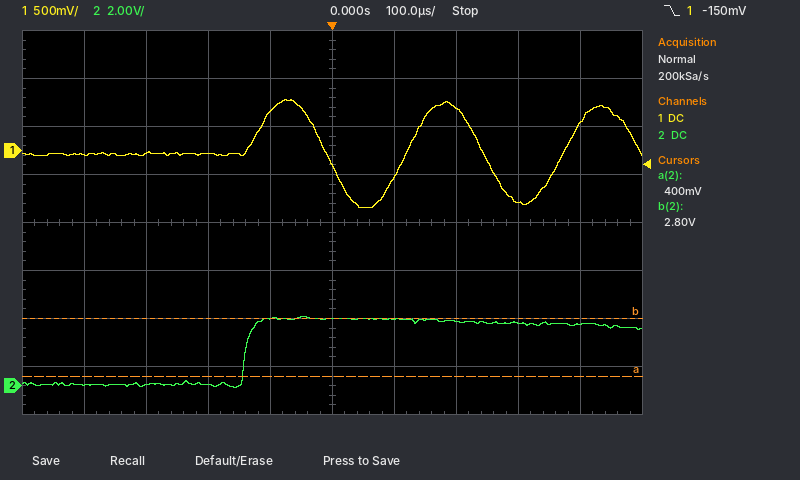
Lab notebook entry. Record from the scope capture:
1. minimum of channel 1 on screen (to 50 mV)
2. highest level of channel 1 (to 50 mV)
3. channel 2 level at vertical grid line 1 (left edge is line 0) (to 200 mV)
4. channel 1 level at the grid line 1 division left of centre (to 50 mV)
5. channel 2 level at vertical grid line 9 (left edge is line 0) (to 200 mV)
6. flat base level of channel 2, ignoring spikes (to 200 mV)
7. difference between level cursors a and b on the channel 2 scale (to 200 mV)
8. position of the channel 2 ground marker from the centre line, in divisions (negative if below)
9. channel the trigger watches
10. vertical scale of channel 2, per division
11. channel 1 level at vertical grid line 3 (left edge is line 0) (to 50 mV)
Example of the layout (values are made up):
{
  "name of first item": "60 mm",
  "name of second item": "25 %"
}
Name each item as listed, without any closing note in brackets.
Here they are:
{
  "minimum of channel 1 on screen": "-600 mV",
  "highest level of channel 1": "550 mV",
  "channel 2 level at vertical grid line 1 (left edge is line 0)": "0.0 V",
  "channel 1 level at the grid line 1 division left of centre": "400 mV",
  "channel 2 level at vertical grid line 9 (left edge is line 0)": "2.6 V",
  "flat base level of channel 2, ignoring spikes": "0.0 V",
  "difference between level cursors a and b on the channel 2 scale": "2.4 V",
  "position of the channel 2 ground marker from the centre line, in divisions": "-3.4 div",
  "channel the trigger watches": "channel 1",
  "vertical scale of channel 2, per division": "2 V",
  "channel 1 level at vertical grid line 3 (left edge is line 0)": "-50 mV"
}
